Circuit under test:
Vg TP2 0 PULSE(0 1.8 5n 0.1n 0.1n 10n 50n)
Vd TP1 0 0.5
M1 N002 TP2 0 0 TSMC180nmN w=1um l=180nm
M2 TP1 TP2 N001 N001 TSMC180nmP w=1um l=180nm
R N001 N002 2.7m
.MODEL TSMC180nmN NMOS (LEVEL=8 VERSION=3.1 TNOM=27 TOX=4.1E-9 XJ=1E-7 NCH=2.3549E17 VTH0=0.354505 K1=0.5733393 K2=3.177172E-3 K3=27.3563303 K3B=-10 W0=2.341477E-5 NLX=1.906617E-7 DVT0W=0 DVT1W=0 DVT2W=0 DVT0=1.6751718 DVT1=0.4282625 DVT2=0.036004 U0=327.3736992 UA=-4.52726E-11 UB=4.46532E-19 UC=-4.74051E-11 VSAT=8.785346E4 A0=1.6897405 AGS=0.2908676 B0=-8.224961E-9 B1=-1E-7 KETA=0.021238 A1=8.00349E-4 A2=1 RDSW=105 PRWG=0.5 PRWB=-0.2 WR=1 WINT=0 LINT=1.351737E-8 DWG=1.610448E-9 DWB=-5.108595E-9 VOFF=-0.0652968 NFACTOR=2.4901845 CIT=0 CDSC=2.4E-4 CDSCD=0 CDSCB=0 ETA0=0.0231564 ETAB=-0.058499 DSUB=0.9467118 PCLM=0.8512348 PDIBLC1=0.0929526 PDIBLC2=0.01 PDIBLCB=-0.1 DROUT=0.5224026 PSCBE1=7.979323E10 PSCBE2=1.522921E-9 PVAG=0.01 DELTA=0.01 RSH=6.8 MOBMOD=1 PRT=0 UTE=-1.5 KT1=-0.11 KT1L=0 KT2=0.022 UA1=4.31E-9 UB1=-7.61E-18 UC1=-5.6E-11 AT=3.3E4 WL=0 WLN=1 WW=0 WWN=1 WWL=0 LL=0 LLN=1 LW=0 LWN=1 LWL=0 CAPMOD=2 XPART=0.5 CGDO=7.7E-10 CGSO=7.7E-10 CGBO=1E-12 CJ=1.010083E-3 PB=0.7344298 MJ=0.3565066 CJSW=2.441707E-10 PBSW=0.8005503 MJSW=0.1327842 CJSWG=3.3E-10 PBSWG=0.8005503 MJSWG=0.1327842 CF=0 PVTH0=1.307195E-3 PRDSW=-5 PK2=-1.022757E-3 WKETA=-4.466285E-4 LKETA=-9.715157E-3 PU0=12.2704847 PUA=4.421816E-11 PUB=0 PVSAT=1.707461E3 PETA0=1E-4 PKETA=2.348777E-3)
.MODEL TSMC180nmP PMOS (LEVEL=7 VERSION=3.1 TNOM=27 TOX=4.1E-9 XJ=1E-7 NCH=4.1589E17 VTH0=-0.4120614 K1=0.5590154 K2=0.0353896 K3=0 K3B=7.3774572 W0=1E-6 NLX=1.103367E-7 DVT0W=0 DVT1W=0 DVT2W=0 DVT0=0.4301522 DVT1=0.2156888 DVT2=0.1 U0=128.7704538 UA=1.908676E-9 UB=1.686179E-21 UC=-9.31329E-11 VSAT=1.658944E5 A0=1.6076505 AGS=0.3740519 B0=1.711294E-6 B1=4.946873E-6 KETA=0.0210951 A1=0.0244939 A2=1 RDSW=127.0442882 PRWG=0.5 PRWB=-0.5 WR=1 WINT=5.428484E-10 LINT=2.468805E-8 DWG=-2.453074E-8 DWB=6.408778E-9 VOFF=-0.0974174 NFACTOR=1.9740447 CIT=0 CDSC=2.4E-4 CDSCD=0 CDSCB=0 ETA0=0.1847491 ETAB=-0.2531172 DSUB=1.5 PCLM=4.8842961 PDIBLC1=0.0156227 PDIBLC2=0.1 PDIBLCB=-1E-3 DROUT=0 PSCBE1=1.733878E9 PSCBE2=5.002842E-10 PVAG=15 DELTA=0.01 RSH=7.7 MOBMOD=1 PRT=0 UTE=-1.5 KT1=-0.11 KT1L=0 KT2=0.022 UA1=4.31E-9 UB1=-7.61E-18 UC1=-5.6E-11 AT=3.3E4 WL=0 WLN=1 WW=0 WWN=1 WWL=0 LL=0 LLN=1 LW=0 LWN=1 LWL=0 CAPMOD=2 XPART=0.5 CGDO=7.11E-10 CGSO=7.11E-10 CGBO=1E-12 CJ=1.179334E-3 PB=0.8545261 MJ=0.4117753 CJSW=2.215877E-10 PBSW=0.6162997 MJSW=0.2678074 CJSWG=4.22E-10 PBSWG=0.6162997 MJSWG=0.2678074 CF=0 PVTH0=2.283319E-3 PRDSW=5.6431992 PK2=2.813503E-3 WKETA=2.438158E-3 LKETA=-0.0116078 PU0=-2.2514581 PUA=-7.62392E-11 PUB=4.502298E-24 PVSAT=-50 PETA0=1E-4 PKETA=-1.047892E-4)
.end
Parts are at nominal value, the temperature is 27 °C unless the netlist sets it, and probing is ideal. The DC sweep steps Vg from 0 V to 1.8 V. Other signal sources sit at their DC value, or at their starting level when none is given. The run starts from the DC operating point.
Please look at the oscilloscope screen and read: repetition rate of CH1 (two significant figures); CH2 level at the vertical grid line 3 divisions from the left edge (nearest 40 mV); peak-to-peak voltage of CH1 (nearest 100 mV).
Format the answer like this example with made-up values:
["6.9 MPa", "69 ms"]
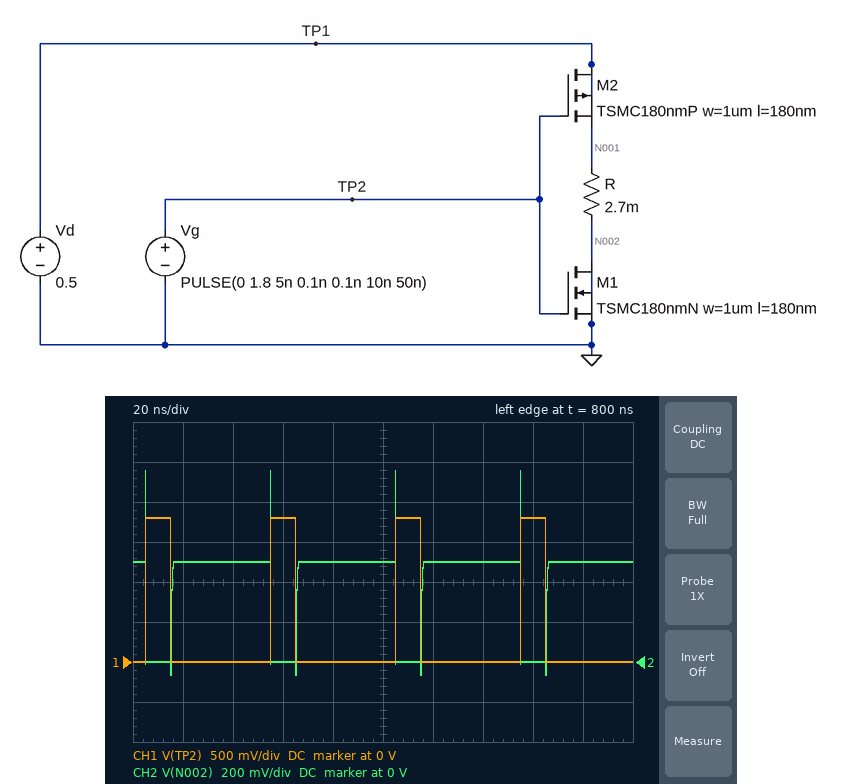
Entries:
["20 MHz", "0 V", "1.8 V"]
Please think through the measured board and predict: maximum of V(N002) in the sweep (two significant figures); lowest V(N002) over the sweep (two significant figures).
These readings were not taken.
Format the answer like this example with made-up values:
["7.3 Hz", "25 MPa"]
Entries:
["500 mV", "1.4 mV"]
